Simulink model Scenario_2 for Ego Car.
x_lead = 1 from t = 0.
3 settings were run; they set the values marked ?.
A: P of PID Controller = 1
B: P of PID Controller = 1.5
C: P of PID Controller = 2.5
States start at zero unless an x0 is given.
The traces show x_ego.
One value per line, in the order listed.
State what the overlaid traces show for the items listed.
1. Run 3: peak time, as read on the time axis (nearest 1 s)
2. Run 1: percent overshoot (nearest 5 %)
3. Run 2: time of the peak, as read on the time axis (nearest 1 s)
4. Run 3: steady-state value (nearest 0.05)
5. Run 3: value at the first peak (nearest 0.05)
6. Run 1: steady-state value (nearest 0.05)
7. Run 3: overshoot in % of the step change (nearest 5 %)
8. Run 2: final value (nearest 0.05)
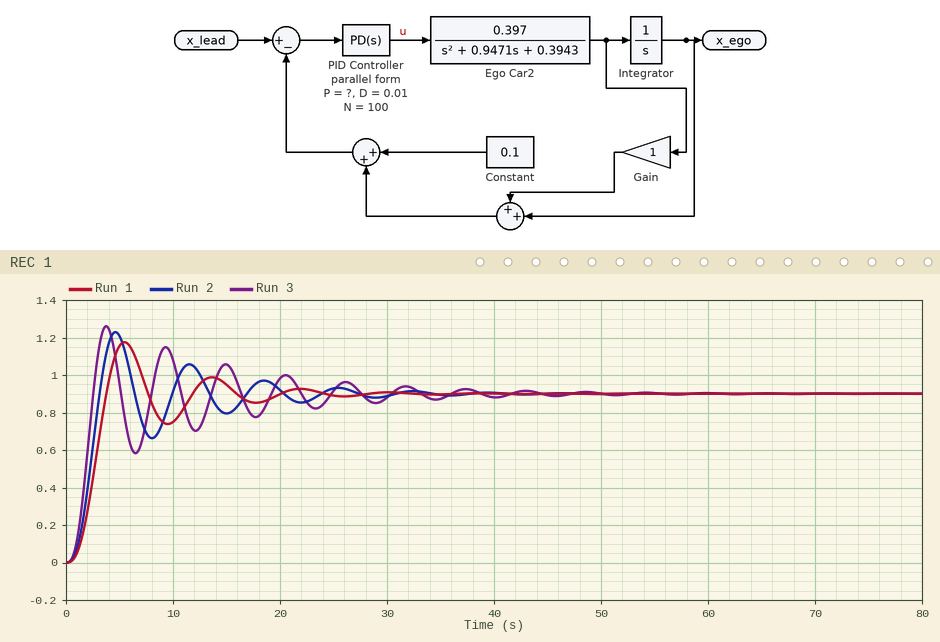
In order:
4 s
30 %
5 s
0.90
1.25
0.90
40 %
0.90
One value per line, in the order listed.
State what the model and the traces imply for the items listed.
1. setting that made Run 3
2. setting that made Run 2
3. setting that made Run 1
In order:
C
B
A
